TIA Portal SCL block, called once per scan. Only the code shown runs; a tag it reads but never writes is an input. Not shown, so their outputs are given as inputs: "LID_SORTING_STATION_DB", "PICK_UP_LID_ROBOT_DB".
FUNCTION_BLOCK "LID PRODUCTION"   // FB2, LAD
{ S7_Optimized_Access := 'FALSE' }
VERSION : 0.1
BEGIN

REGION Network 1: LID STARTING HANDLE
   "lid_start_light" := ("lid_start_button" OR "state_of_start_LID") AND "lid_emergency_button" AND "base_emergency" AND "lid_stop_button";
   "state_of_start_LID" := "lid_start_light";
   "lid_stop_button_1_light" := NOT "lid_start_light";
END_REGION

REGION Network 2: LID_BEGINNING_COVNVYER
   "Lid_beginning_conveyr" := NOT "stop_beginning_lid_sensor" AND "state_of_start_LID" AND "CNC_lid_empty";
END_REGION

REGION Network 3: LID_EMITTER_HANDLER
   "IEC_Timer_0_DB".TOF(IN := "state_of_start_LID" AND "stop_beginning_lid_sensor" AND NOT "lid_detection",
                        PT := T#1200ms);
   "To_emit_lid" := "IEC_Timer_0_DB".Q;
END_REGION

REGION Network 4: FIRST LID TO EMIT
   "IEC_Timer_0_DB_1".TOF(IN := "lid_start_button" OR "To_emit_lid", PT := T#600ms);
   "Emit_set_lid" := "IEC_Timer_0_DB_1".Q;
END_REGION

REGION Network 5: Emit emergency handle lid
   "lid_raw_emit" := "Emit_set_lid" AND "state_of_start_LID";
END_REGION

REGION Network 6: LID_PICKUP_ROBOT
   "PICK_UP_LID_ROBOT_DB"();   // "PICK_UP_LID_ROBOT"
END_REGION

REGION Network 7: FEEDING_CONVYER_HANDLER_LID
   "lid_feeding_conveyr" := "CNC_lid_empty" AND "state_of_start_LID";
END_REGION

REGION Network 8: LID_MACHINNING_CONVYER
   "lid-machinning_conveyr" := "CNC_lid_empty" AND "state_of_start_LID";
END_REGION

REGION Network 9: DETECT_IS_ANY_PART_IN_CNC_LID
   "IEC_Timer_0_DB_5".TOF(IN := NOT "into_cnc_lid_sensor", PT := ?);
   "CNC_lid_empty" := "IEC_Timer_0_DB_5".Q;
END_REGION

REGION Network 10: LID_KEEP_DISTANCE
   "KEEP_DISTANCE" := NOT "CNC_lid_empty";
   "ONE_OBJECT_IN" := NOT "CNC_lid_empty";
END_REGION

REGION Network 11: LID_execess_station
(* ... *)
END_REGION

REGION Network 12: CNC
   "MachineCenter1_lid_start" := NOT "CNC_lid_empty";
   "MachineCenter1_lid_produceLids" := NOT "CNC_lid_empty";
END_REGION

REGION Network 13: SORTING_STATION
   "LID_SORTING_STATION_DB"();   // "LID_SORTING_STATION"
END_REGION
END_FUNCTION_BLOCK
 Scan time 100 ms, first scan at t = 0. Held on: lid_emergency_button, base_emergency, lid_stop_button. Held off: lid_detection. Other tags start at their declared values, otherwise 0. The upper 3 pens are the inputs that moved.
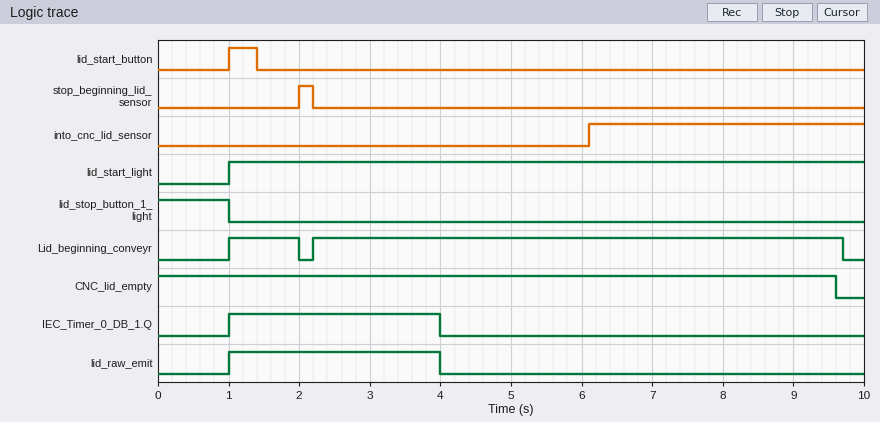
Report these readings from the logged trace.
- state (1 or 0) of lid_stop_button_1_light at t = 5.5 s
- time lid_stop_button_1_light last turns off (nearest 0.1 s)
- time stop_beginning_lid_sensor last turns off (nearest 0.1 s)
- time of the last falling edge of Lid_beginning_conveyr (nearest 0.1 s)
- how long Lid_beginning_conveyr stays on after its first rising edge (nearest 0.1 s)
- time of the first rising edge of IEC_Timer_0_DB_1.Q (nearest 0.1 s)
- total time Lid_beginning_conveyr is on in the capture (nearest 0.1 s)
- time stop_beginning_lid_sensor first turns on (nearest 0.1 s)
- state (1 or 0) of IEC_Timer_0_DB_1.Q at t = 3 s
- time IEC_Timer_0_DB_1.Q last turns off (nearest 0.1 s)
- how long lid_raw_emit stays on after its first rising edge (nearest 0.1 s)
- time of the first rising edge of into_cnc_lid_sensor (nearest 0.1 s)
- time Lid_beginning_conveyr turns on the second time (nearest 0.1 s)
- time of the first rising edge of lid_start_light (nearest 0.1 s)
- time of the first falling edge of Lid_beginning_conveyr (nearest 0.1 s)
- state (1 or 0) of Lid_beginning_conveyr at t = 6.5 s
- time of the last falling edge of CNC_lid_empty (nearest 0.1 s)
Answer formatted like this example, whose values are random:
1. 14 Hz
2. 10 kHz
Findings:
1. 0
2. 1.0 s
3. 2.2 s
4. 9.7 s
5. 1.0 s
6. 1.0 s
7. 8.5 s
8. 2.0 s
9. 1
10. 4.0 s
11. 3.0 s
12. 6.1 s
13. 2.2 s
14. 1.0 s
15. 2.0 s
16. 1
17. 9.6 s
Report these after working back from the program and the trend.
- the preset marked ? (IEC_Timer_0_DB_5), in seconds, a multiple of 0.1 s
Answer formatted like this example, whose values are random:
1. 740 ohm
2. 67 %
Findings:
1. 3.5 s
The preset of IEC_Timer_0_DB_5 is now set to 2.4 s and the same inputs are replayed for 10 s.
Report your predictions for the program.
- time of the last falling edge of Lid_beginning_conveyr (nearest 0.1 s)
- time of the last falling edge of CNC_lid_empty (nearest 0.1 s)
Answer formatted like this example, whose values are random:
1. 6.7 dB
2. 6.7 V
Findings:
1. 8.6 s
2. 8.5 s
